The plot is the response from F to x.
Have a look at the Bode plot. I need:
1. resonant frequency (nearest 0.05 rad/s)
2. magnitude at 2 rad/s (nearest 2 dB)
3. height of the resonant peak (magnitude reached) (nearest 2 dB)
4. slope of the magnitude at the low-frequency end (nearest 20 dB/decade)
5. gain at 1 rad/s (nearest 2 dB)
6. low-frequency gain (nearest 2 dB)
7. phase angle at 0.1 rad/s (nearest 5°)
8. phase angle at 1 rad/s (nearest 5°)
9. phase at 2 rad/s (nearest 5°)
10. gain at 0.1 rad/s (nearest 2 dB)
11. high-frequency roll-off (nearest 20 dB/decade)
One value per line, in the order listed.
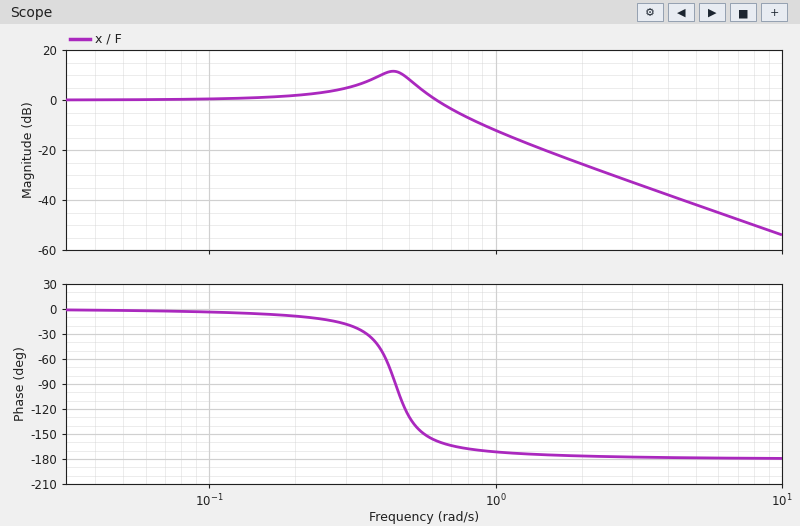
0.45 rad/s
-26 dB
12 dB
0 dB/decade
-12 dB
0 dB
-5°
-170°
-175°
0 dB
-40 dB/decade
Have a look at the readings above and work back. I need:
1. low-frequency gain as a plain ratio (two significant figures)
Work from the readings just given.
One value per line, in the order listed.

1.0
